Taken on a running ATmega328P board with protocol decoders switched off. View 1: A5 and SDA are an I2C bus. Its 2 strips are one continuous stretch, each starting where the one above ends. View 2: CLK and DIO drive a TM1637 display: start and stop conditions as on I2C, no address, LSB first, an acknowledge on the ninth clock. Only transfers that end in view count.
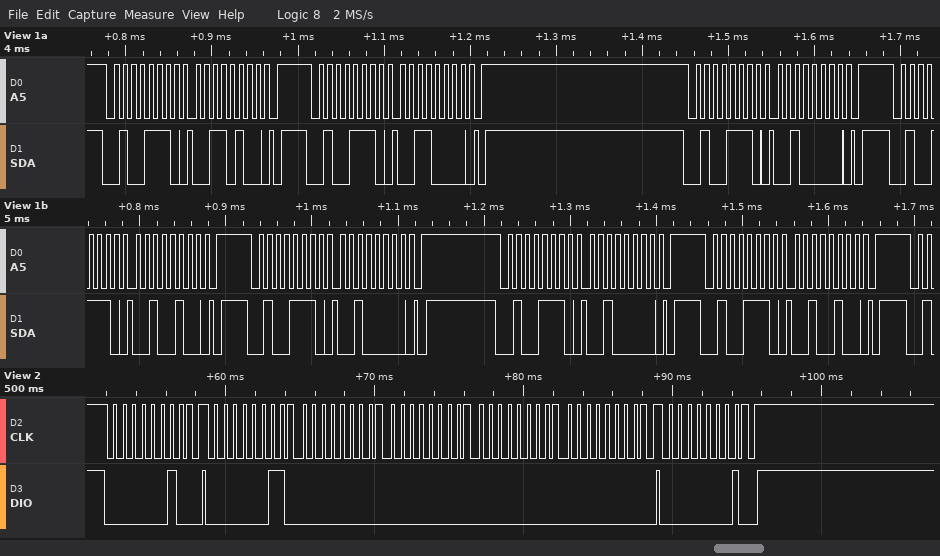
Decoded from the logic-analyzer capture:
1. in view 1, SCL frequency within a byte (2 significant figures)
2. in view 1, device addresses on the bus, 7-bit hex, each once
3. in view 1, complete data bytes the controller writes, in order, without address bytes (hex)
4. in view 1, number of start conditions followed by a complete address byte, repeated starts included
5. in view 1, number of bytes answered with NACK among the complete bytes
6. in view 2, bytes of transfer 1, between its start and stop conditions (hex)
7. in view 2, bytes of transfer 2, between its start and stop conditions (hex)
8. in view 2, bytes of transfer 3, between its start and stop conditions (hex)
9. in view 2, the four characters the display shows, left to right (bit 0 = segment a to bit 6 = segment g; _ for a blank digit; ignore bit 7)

100 kHz
0x27
34 30 20 24 20 20 24
7
0
40
C0 00 00 00 00
80
____
